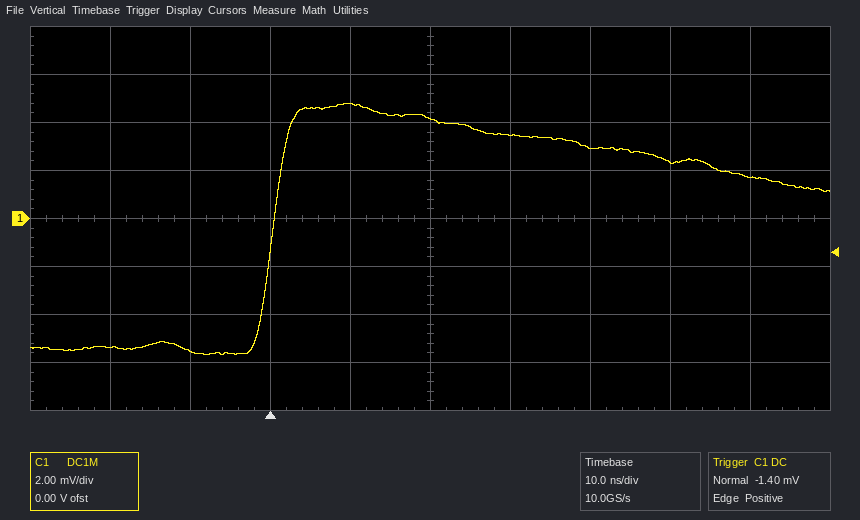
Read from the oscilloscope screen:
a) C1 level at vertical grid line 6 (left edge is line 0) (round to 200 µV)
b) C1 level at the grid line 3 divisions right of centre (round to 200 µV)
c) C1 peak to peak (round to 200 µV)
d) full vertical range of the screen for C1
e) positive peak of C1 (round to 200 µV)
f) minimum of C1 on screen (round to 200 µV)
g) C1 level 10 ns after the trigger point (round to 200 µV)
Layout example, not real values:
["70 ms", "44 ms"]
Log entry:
["3.4 mV", "2.4 mV", "10.4 mV", "16 mV", "4.8 mV", "-5.6 mV", "4.8 mV"]
